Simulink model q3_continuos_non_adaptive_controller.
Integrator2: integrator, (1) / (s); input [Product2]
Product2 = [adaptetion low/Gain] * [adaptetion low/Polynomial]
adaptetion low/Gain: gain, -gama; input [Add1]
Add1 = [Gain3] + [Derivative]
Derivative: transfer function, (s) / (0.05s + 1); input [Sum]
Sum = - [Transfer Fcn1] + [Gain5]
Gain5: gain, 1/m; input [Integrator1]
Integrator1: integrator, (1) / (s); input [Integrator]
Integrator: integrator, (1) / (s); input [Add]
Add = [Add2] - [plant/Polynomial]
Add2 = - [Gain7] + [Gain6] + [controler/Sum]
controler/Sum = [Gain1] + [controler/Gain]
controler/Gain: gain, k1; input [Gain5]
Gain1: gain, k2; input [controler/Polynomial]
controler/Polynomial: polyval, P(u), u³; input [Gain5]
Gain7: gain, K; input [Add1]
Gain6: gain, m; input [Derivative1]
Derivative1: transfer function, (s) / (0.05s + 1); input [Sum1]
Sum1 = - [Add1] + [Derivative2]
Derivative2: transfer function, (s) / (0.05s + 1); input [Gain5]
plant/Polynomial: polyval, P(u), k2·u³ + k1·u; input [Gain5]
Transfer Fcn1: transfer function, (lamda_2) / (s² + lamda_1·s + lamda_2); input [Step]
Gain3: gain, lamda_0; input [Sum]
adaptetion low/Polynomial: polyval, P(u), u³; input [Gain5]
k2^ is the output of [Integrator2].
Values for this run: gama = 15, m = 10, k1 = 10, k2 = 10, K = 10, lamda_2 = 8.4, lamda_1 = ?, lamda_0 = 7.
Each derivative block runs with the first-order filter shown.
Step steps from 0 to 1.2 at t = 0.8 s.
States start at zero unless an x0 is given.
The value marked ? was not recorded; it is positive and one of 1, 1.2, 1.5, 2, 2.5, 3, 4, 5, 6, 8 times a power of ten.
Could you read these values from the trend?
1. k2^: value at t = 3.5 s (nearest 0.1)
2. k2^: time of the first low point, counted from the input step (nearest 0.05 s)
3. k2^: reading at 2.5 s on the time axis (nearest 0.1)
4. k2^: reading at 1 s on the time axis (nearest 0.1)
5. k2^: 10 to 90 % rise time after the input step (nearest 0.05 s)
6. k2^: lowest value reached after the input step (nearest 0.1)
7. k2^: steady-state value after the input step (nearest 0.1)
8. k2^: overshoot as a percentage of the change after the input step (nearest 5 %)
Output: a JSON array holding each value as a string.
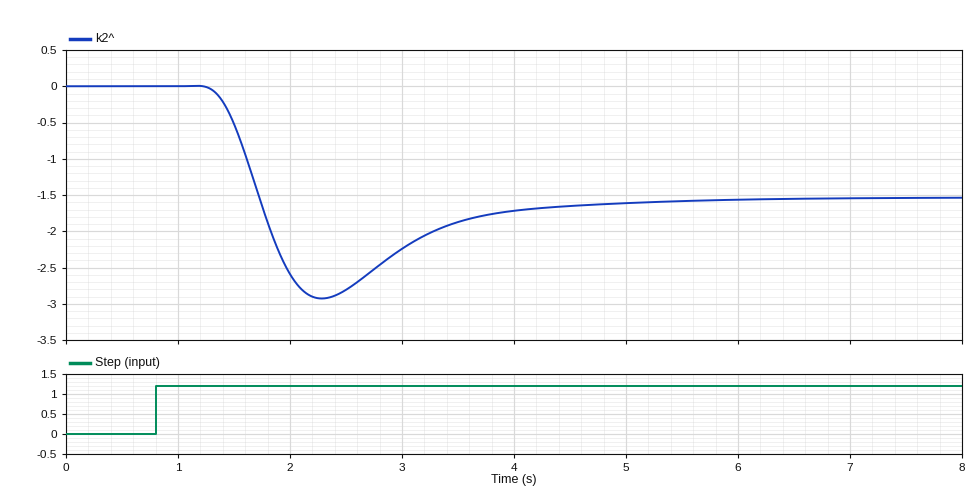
["-1.9", "1.50 s", "-2.8", "0.0", "0.30 s", "-2.9", "-1.5", "90 %"]
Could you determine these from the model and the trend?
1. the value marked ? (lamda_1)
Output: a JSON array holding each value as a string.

["4"]
